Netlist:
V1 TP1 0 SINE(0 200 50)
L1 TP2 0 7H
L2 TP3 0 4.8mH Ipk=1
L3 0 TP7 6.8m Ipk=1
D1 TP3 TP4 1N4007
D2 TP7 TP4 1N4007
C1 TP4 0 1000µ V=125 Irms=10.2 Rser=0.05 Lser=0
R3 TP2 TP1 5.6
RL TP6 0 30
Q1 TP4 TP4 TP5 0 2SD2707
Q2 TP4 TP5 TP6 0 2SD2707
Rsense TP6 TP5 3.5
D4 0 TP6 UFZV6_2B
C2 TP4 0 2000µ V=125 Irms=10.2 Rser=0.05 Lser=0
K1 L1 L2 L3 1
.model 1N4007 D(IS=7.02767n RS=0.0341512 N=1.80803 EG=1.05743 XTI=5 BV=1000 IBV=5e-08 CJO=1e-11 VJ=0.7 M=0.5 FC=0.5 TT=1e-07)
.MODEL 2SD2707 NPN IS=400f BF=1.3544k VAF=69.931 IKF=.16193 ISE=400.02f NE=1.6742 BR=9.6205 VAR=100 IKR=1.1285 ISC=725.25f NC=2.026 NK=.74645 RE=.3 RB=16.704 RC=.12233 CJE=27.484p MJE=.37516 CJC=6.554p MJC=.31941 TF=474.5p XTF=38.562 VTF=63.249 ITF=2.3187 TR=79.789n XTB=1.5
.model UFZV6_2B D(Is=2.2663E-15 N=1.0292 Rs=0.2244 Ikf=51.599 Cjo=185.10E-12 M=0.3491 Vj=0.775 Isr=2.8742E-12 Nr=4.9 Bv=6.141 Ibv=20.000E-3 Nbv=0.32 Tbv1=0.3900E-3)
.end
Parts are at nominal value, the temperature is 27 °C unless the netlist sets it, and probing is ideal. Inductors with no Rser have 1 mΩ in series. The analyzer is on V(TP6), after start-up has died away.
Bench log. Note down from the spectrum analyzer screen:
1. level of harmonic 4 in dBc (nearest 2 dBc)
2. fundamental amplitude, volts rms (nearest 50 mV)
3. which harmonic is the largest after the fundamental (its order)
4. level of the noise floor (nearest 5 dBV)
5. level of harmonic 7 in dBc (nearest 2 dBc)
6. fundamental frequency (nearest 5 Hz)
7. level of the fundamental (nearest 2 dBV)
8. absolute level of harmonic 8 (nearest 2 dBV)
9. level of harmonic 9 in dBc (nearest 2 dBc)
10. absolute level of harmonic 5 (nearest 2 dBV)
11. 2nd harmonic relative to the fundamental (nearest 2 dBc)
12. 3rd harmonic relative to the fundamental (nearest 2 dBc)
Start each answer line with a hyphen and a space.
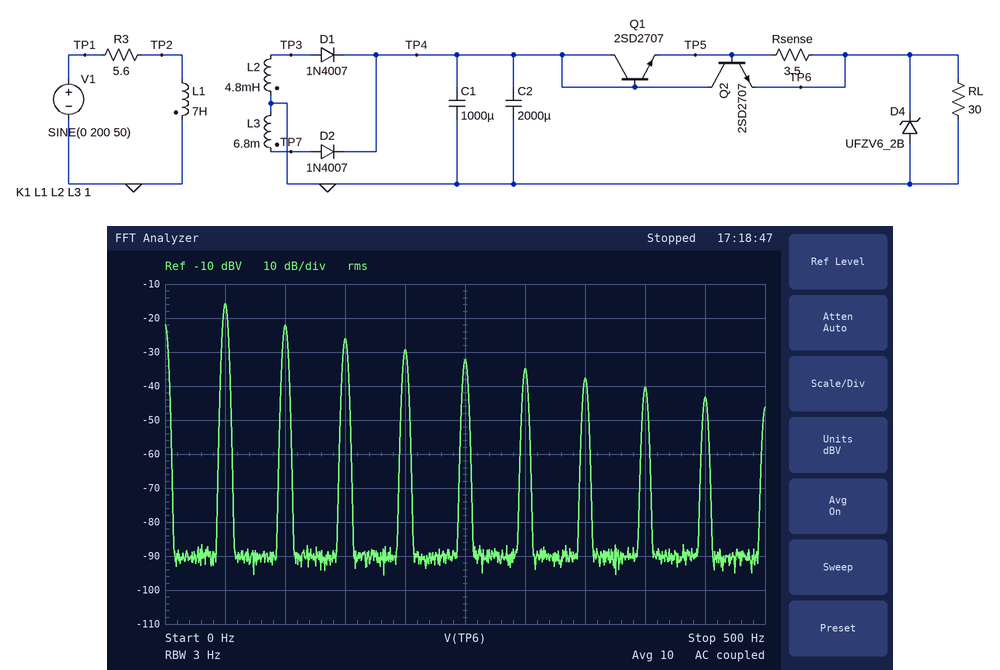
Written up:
- -14 dBc
- 150 mV
- 2
- -90 dBV
- -22 dBc
- 50 Hz
- -16 dBV
- -40 dBV
- -28 dBc
- -32 dBV
- -6 dBc
- -10 dBc
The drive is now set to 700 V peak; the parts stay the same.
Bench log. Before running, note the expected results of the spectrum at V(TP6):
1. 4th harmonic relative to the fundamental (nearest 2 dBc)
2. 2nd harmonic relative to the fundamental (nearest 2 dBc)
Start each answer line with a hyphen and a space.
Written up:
- -10 dBc
- 0 dBc
